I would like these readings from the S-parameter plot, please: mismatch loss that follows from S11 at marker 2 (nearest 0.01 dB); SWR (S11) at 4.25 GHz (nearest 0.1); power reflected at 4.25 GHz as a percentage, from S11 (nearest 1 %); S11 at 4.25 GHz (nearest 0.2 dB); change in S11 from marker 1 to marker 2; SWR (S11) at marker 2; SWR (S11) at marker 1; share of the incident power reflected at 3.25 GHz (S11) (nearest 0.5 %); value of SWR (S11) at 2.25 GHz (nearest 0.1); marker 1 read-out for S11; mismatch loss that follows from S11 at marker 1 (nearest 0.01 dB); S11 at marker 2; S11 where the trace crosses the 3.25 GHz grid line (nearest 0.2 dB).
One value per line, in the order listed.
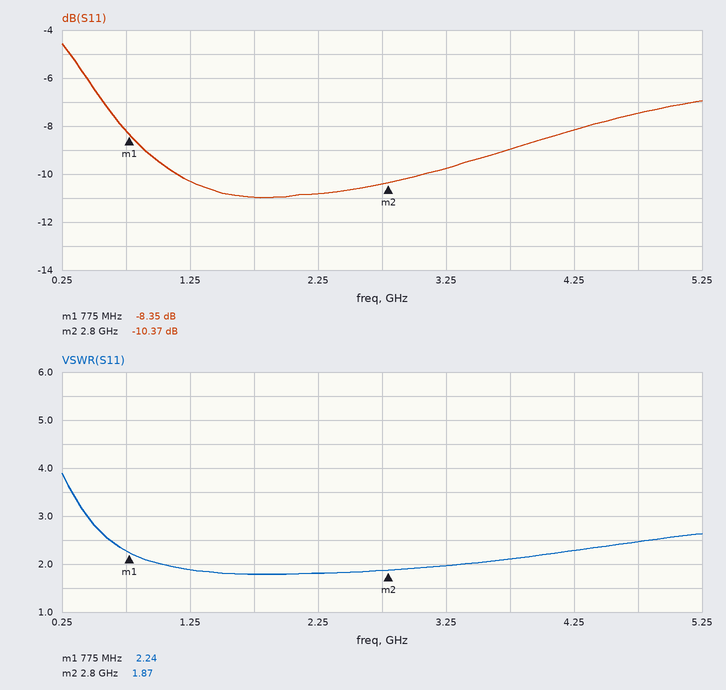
0.42 dB
2.3
15 %
-8.2 dB
-2.02 dB
1.87
2.24
10.5 %
1.8
-8.35 dB
0.69 dB
-10.37 dB
-9.8 dB
